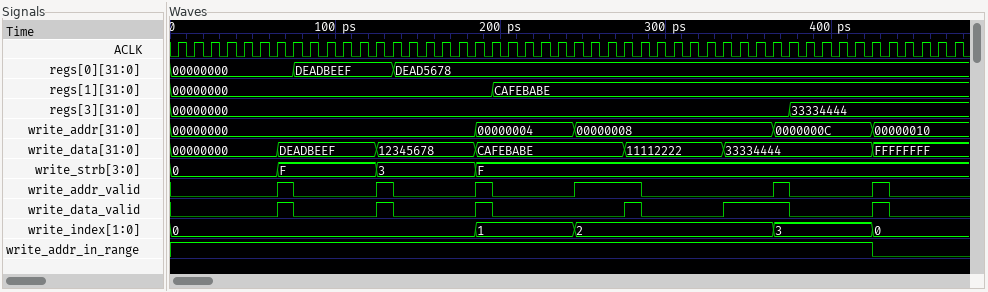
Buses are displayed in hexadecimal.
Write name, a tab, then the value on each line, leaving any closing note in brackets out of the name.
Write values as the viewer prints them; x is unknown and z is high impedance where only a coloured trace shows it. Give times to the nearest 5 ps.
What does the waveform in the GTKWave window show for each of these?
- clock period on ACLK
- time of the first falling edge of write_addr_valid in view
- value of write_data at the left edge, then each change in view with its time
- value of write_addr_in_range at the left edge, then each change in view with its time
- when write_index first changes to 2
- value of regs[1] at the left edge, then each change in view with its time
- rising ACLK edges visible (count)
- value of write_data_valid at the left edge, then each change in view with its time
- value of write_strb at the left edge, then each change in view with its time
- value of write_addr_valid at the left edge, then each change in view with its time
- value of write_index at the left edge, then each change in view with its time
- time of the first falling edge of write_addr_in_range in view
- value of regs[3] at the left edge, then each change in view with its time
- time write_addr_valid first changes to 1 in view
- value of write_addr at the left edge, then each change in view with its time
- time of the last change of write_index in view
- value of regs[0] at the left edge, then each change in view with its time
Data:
clock period on ACLK	10 ps
time of the first falling edge of write_addr_valid in view	75 ps
value of write_data at the left edge, then each change in view with its time	00000000, DEADBEEF at 65 ps, 12345678 at 125 ps, CAFEBABE at 185 ps, 11112222 at 275 ps, 33334444 at 335 ps, FFFFFFFF at 425 ps
value of write_addr_in_range at the left edge, then each change in view with its time	1, 0 at 425 ps
when write_index first changes to 2	245 ps
value of regs[1] at the left edge, then each change in view with its time	00000000, CAFEBABE at 195 ps
rising ACLK edges visible	48
value of write_data_valid at the left edge, then each change in view with its time	0, 1 at 65 ps, 0 at 75 ps, 1 at 125 ps, 0 at 135 ps, 1 at 185 ps, 0 at 195 ps, 1 at 275 ps, 0 at 285 ps, 1 at 335 ps, 0 at 375 ps, 1 at 425 ps, 0 at 435 ps
value of write_strb at the left edge, then each change in view with its time	0, F at 65 ps, 3 at 125 ps, F at 185 ps
value of write_addr_valid at the left edge, then each change in view with its time	0, 1 at 65 ps, 0 at 75 ps, 1 at 125 ps, 0 at 135 ps, 1 at 185 ps, 0 at 195 ps, 1 at 245 ps, 0 at 285 ps, 1 at 365 ps, 0 at 375 ps, 1 at 425 ps, 0 at 435 ps
value of write_index at the left edge, then each change in view with its time	0, 1 at 185 ps, 2 at 245 ps, 3 at 365 ps, 0 at 425 ps
time of the first falling edge of write_addr_in_range in view	425 ps
value of regs[3] at the left edge, then each change in view with its time	00000000, 33334444 at 375 ps
time write_addr_valid first changes to 1 in view	65 ps
value of write_addr at the left edge, then each change in view with its time	00000000, 00000004 at 185 ps, 00000008 at 245 ps, 0000000C at 365 ps, 00000010 at 425 ps
time of the last change of write_index in view	425 ps
value of regs[0] at the left edge, then each change in view with its time	00000000, DEADBEEF at 75 ps, DEAD5678 at 135 ps
